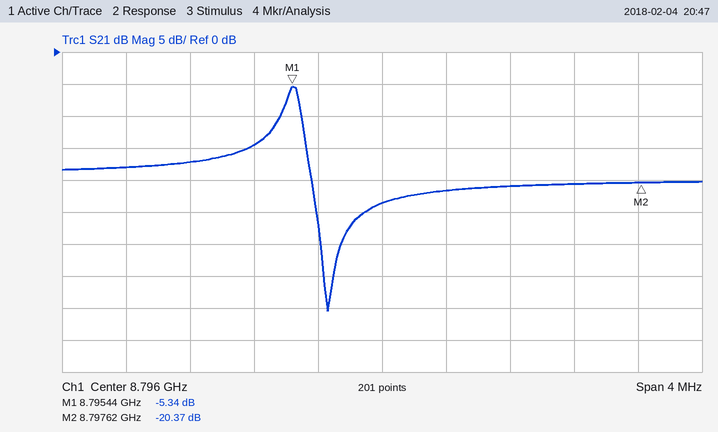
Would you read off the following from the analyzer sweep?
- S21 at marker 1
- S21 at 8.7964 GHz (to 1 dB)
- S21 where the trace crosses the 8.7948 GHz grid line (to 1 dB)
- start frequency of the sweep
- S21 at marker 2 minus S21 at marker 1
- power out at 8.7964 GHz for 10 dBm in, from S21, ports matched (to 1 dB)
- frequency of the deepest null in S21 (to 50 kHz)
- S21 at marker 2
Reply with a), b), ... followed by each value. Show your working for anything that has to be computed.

a) -5.34 dB
b) -22 dB
c) -17 dB
d) 8.794 GHz
e) -20.37 − (-5.34) = -15.03 dB
f) 10 dBm + (-22 dB) = -12 dBm
g) 8.79565 GHz
h) -20.37 dB
